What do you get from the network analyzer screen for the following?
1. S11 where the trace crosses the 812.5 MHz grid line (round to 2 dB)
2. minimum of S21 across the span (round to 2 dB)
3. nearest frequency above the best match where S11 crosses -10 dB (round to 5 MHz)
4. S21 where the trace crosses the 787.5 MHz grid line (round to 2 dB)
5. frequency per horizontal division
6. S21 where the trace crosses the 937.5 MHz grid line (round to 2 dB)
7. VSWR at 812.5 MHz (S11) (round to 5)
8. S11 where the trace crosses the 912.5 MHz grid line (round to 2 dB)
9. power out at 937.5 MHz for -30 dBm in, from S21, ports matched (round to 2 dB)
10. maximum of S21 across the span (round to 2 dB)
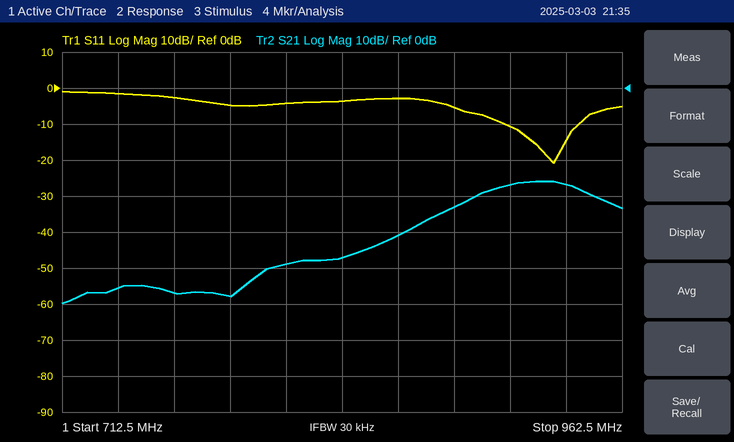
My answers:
-4 dB
-60 dB
945 MHz
-58 dB
25 MHz
-26 dB
5
-10 dB
-56 dBm
-26 dB
